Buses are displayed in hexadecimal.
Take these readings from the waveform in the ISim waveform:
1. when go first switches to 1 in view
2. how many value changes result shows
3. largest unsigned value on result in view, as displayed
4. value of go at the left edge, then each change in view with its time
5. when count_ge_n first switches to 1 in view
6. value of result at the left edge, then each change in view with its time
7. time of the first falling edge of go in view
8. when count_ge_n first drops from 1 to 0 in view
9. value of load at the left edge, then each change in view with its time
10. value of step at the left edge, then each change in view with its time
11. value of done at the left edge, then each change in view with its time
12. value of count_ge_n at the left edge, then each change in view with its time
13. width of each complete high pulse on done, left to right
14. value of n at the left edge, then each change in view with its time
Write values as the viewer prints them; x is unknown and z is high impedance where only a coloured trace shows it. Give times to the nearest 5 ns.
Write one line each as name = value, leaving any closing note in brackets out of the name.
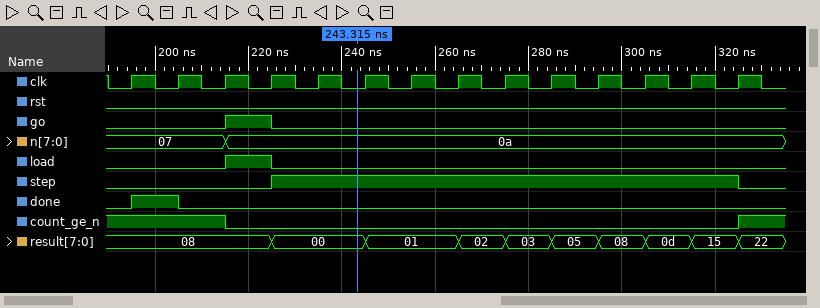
when go first switches to 1 in view = 215 ns
how many value changes result shows = 9
largest unsigned value on result in view, as displayed = 22
value of go at the left edge, then each change in view with its time = 0, 1 at 215 ns, 0 at 225 ns
when count_ge_n first switches to 1 in view = 325 ns
value of result at the left edge, then each change in view with its time = 08, 00 at 225 ns, 01 at 245 ns, 02 at 265 ns, 03 at 275 ns, 05 at 285 ns, 08 at 295 ns, 0d at 305 ns, 15 at 315 ns, 22 at 325 ns
time of the first falling edge of go in view = 225 ns
when count_ge_n first drops from 1 to 0 in view = 215 ns
value of load at the left edge, then each change in view with its time = 0, 1 at 215 ns, 0 at 225 ns
value of step at the left edge, then each change in view with its time = 0, 1 at 225 ns, 0 at 325 ns
value of done at the left edge, then each change in view with its time = 0, 1 at 195 ns, 0 at 205 ns
value of count_ge_n at the left edge, then each change in view with its time = 1, 0 at 215 ns, 1 at 325 ns
width of each complete high pulse on done, left to right = 10 ns
value of n at the left edge, then each change in view with its time = 07, 0a at 215 ns
